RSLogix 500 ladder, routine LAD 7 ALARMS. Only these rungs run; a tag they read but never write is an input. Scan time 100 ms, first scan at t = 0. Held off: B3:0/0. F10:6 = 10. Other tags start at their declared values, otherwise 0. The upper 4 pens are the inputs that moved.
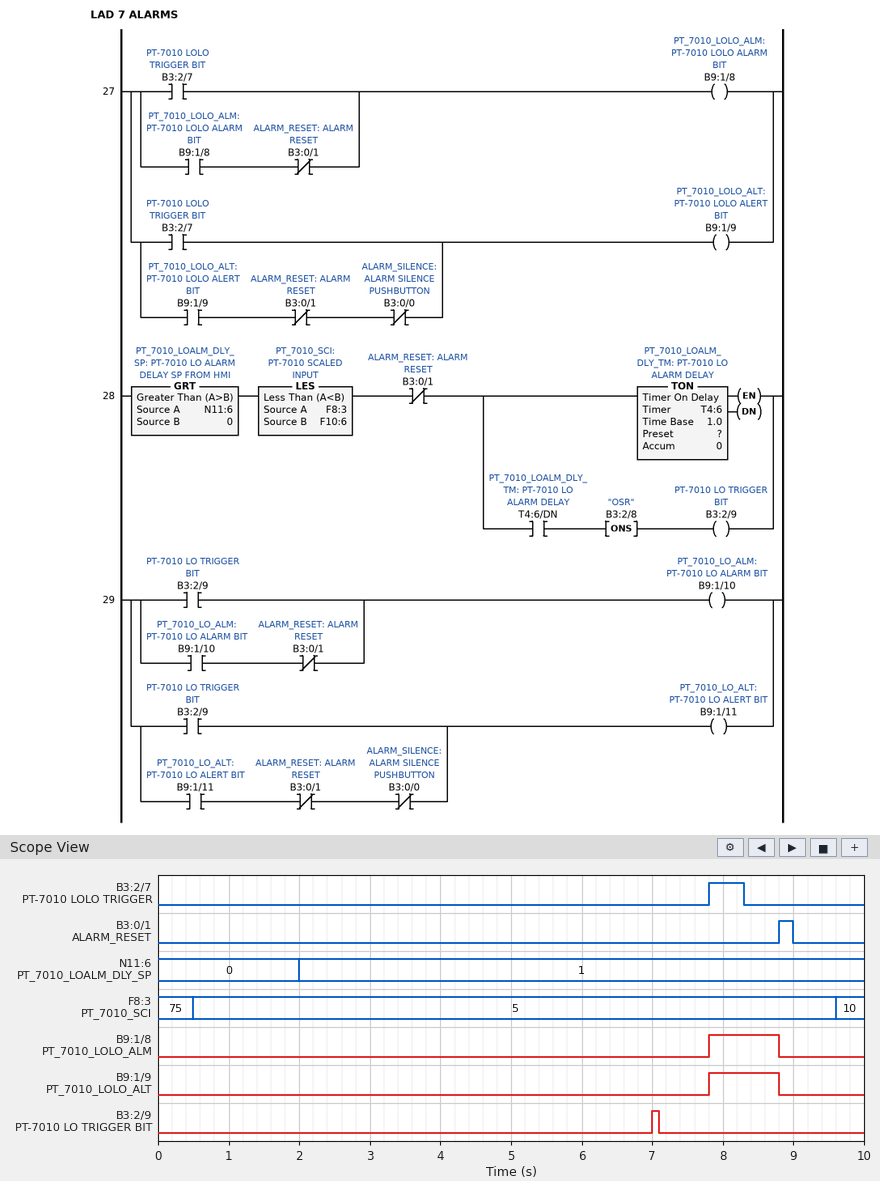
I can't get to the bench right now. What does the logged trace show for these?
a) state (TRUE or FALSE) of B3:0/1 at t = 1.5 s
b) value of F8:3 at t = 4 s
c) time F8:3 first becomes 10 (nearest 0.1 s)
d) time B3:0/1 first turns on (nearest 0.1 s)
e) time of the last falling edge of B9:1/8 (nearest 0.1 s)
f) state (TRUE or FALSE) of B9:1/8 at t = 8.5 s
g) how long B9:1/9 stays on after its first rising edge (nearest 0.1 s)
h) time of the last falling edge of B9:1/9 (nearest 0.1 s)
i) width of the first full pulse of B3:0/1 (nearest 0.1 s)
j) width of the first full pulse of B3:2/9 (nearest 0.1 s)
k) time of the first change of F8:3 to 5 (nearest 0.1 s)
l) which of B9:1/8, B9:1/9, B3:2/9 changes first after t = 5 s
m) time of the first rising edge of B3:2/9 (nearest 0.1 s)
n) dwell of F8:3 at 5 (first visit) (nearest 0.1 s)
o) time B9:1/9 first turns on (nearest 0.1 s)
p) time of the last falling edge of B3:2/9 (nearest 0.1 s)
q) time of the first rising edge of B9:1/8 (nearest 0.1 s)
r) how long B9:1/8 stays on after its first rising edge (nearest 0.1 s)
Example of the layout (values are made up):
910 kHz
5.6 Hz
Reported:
FALSE
5
9.6 s
8.8 s
8.8 s
TRUE
1.0 s
8.8 s
0.2 s
0.1 s
0.5 s
B3:2/9
7.0 s
9.1 s
7.8 s
7.1 s
7.8 s
1.0 s
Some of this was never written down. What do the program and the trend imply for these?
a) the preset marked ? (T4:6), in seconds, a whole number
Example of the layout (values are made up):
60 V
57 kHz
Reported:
5 s
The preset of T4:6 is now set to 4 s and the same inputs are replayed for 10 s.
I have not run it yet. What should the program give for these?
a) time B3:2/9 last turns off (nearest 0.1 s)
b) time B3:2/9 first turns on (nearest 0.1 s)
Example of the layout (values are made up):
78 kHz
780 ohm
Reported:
6.1 s
6.0 s
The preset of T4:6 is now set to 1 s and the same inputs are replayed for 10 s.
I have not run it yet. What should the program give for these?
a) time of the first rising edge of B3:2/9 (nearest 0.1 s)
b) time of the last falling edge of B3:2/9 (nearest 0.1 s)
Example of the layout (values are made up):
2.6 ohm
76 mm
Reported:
3.0 s
3.1 s
